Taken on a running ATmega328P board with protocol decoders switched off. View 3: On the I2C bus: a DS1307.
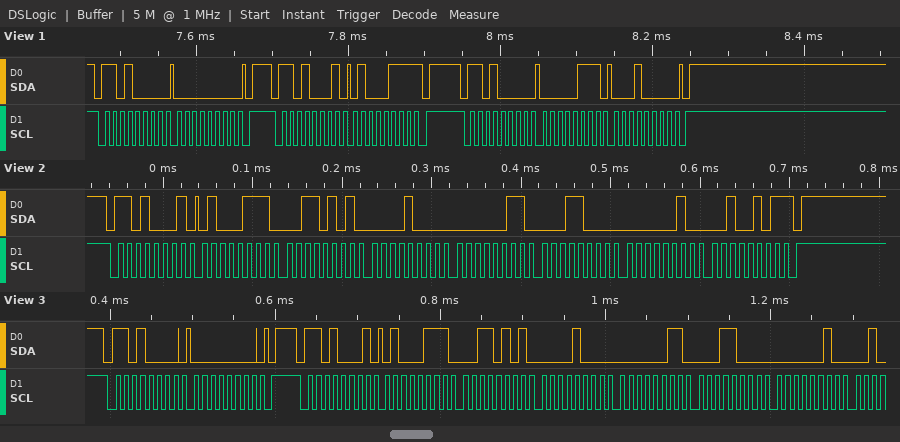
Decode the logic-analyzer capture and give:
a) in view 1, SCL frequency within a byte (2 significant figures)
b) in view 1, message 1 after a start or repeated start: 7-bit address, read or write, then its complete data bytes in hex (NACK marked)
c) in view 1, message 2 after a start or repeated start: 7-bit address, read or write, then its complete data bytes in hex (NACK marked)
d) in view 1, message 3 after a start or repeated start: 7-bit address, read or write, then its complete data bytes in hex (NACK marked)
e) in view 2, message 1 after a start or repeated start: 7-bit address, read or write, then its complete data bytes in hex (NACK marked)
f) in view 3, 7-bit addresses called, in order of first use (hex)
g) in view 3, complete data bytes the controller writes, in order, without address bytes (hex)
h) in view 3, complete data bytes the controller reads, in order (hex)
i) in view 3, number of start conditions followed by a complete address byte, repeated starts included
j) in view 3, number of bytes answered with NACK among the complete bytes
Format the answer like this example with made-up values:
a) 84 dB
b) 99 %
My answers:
a) 100 kHz
b) 0x68 write: 00
c) 0x68 read: 47 NACK
d) 0x68 write: 07 10
e) 0x68 read: 47 35 08 03 18 02 25 NACK
f) 0x68
g) 00
h) 47 35 08 03 18 02
i) 2
j) 0
